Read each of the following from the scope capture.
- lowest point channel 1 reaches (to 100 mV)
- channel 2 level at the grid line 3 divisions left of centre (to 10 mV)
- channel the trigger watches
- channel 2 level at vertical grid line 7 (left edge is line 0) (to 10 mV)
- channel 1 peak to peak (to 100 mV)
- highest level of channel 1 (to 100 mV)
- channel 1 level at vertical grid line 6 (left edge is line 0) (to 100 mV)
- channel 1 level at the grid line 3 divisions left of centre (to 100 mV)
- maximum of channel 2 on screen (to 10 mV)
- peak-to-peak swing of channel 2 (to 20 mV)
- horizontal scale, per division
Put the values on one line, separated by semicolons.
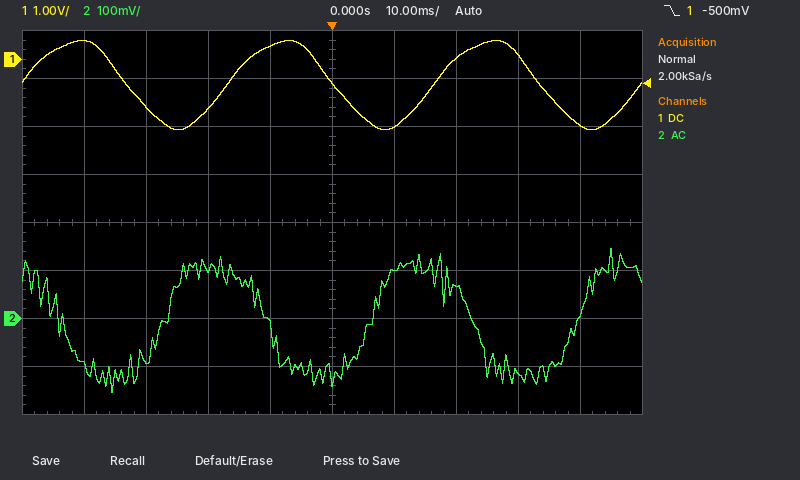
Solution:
-1.5 V; -90 mV; channel 1; 70 mV; 1.9 V; 400 mV; -1.4 V; -1.0 V; 150 mV; 300 mV; 10 ms
